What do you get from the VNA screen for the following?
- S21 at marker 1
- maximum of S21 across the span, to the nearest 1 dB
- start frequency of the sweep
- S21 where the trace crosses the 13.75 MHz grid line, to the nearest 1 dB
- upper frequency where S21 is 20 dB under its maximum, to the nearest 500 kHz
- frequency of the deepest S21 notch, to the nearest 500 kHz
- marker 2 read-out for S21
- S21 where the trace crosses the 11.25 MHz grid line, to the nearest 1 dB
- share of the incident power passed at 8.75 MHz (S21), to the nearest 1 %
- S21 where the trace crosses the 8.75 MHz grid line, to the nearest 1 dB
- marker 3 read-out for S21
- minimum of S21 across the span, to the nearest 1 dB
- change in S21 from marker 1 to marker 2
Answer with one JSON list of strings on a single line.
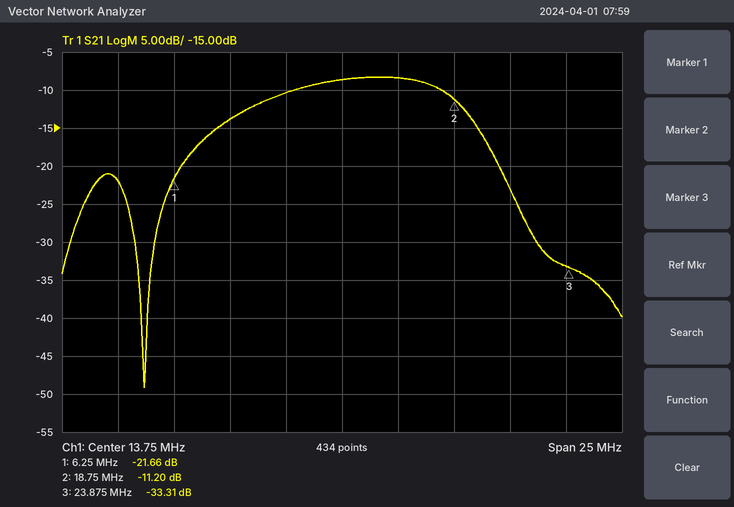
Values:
["-21.66 dB", "-8 dB", "1.25 MHz", "-9 dB", "22.0 MHz", "5.0 MHz", "-11.20 dB", "-10 dB", "4 %", "-14 dB", "-33.31 dB", "-49 dB", "10.46 dB"]
